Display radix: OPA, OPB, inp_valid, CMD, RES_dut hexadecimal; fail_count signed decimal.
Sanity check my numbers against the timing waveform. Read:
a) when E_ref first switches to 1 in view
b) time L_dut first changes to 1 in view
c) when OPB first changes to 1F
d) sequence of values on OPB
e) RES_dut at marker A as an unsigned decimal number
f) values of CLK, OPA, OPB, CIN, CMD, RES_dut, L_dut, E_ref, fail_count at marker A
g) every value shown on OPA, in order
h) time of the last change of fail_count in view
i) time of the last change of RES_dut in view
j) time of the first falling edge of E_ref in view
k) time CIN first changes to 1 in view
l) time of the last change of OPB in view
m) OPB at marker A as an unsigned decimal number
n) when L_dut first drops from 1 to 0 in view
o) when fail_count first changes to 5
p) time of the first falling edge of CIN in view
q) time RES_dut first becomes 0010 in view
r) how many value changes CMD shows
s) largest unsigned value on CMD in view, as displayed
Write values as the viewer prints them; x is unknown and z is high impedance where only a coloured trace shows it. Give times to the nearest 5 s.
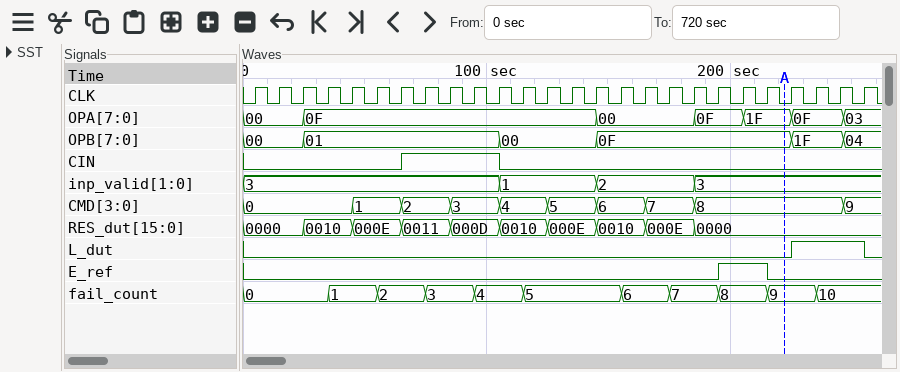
195 s
225 s
225 s
00, 01, 00, 0F, 1F, 04
0
CLK=0, OPA=1F, OPB=0F, CIN=0, CMD=8, RES_dut=0000, L_dut=0, E_ref=0, fail_count=9
00, 0F, 00, 0F, 1F, 0F, 03
235 s
185 s
215 s
65 s
245 s
15
255 s
115 s
105 s
25 s
9
9
